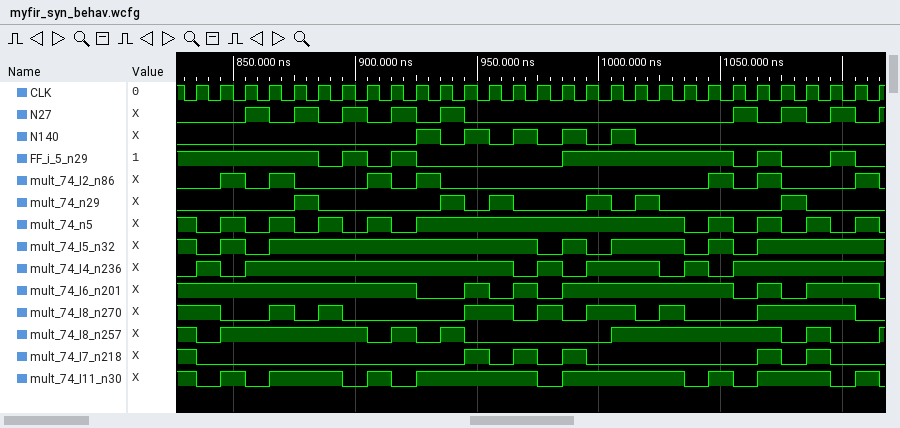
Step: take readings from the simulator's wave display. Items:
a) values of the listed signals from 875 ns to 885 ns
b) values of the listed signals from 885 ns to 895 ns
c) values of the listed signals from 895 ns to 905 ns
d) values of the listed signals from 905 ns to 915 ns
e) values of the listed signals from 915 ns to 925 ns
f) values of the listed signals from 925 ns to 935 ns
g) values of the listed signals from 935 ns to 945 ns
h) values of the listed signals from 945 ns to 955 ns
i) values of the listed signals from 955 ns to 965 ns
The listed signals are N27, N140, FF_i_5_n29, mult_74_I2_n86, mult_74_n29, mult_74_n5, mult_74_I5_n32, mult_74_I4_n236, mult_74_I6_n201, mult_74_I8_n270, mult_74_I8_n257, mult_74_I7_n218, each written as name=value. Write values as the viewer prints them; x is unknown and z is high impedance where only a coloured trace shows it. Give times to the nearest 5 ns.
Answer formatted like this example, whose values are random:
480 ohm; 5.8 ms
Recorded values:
N27=1, N140=0, FF_i_5_n29=1, mult_74_I2_n86=0, mult_74_n29=1, mult_74_n5=0, mult_74_I5_n32=1, mult_74_I4_n236=1, mult_74_I6_n201=1, mult_74_I8_n270=0, mult_74_I8_n257=1, mult_74_I7_n218=0; N27=0, N140=0, FF_i_5_n29=0, mult_74_I2_n86=0, mult_74_n29=0, mult_74_n5=1, mult_74_I5_n32=1, mult_74_I4_n236=1, mult_74_I6_n201=1, mult_74_I8_n270=1, mult_74_I8_n257=1, mult_74_I7_n218=0; N27=1, N140=0, FF_i_5_n29=1, mult_74_I2_n86=0, mult_74_n29=0, mult_74_n5=0, mult_74_I5_n32=1, mult_74_I4_n236=1, mult_74_I6_n201=1, mult_74_I8_n270=0, mult_74_I8_n257=1, mult_74_I7_n218=0; N27=0, N140=0, FF_i_5_n29=0, mult_74_I2_n86=1, mult_74_n29=0, mult_74_n5=1, mult_74_I5_n32=1, mult_74_I4_n236=1, mult_74_I6_n201=1, mult_74_I8_n270=0, mult_74_I8_n257=0, mult_74_I7_n218=0; N27=1, N140=0, FF_i_5_n29=1, mult_74_I2_n86=0, mult_74_n29=0, mult_74_n5=0, mult_74_I5_n32=1, mult_74_I4_n236=1, mult_74_I6_n201=1, mult_74_I8_n270=0, mult_74_I8_n257=1, mult_74_I7_n218=0; N27=0, N140=1, FF_i_5_n29=0, mult_74_I2_n86=1, mult_74_n29=0, mult_74_n5=1, mult_74_I5_n32=1, mult_74_I4_n236=1, mult_74_I6_n201=0, mult_74_I8_n270=0, mult_74_I8_n257=0, mult_74_I7_n218=0; N27=1, N140=0, FF_i_5_n29=0, mult_74_I2_n86=0, mult_74_n29=1, mult_74_n5=1, mult_74_I5_n32=1, mult_74_I4_n236=1, mult_74_I6_n201=0, mult_74_I8_n270=0, mult_74_I8_n257=1, mult_74_I7_n218=0; N27=0, N140=1, FF_i_5_n29=0, mult_74_I2_n86=0, mult_74_n29=0, mult_74_n5=1, mult_74_I5_n32=1, mult_74_I4_n236=1, mult_74_I6_n201=1, mult_74_I8_n270=1, mult_74_I8_n257=0, mult_74_I7_n218=1; N27=0, N140=0, FF_i_5_n29=0, mult_74_I2_n86=0, mult_74_n29=1, mult_74_n5=1, mult_74_I5_n32=1, mult_74_I4_n236=1, mult_74_I6_n201=0, mult_74_I8_n270=1, mult_74_I8_n257=0, mult_74_I7_n218=0
